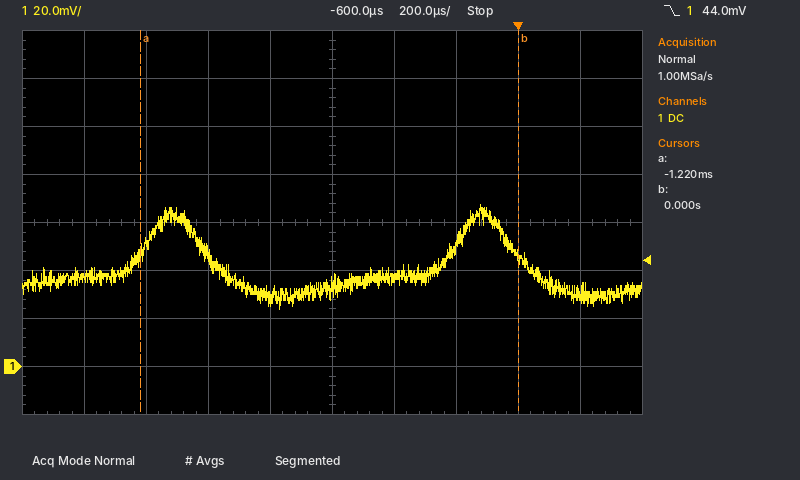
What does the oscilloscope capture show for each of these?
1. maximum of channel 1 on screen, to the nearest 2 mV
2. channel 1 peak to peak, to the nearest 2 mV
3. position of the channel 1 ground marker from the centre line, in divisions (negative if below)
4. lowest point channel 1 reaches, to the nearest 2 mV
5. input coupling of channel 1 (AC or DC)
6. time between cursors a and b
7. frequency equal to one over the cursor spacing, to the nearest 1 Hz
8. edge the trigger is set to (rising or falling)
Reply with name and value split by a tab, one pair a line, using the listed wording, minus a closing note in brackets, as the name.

maximum of channel 1 on screen, to the nearest 2 mV	68 mV
channel 1 peak to peak, to the nearest 2 mV	44 mV
position of the channel 1 ground marker from the centre line, in divisions	-3.0 div
lowest point channel 1 reaches, to the nearest 2 mV	24 mV
input coupling of channel 1	DC
time between cursors a and b	1.22 ms
frequency equal to one over the cursor spacing, to the nearest 1 Hz	820 Hz
edge the trigger is set to	falling
